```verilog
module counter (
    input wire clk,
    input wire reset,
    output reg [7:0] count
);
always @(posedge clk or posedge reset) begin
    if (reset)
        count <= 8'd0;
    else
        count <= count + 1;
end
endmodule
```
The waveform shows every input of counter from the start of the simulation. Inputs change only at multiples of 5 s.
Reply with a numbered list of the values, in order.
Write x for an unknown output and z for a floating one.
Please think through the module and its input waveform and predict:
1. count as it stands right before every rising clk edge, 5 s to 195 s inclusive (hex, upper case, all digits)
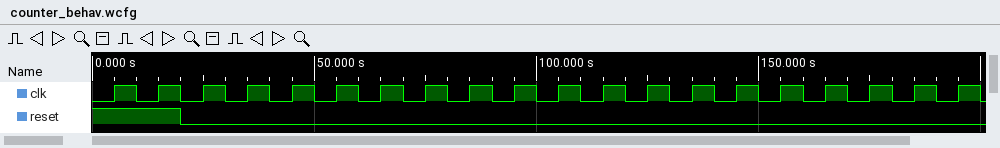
1. 00, 00, 00, 01, 02, 03, 04, 05, 06, 07, 08, 09, 0A, 0B, 0C, 0D, 0E, 0F, 10, 11
